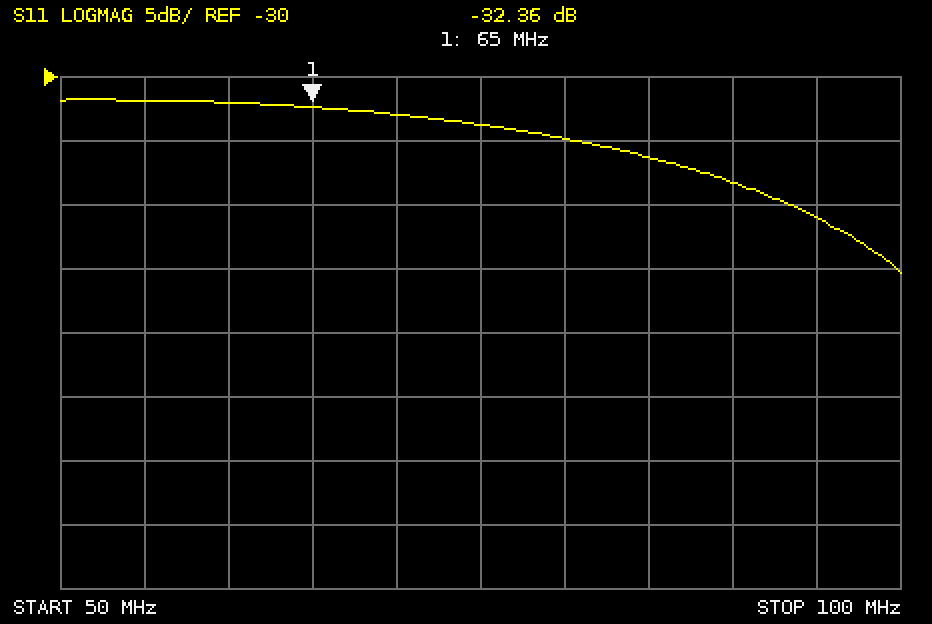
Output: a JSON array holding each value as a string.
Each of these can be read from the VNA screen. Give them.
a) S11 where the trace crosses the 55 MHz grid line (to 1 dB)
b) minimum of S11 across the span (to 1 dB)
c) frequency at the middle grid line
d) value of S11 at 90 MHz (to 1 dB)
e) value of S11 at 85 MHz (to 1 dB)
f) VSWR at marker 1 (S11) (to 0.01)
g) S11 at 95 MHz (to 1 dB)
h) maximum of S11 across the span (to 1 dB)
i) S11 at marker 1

["-32 dB", "-45 dB", "75 MHz", "-38 dB", "-36 dB", "1.05", "-41 dB", "-32 dB", "-32.36 dB"]
